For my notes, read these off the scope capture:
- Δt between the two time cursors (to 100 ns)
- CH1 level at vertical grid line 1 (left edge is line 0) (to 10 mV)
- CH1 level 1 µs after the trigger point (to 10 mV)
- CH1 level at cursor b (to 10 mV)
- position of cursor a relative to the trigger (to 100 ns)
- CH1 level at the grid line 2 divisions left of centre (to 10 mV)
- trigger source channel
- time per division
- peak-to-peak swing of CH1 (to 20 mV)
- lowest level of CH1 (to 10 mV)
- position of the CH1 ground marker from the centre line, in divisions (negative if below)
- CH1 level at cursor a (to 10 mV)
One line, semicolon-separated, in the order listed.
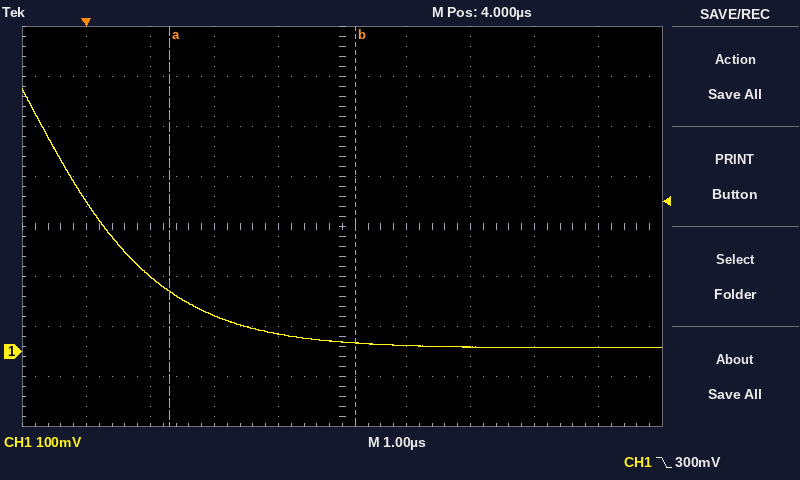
2.9 µs; 300 mV; 150 mV; 20 mV; +1.3 µs; 70 mV; CH1; 1 µs; 520 mV; 10 mV; -2.5 div; 120 mV
